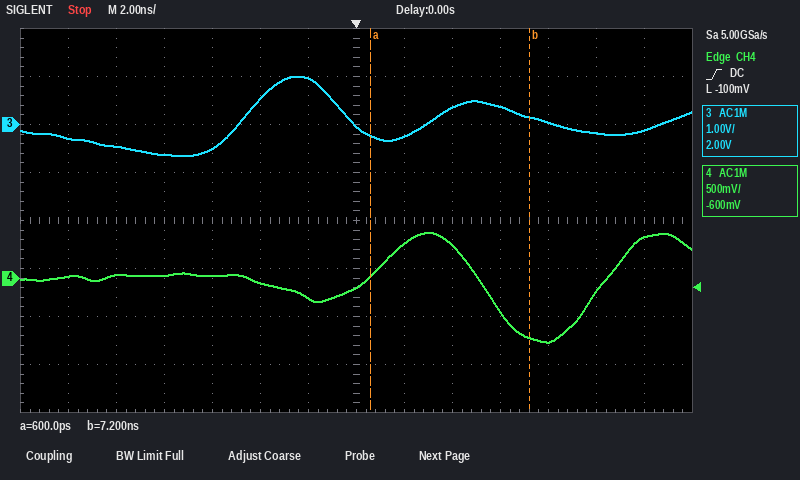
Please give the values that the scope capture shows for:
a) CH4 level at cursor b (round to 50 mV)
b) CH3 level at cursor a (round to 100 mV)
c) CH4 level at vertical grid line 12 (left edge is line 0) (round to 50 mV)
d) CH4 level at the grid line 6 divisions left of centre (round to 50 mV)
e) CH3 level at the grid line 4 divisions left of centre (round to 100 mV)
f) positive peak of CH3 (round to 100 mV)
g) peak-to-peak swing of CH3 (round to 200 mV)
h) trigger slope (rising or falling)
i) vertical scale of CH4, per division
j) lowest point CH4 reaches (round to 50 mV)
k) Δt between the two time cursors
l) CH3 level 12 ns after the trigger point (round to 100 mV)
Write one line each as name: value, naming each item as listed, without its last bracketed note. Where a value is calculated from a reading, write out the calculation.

CH4 level at cursor b: -600 mV
CH3 level at cursor a: -200 mV
CH4 level at vertical grid line 12 (left edge is line 0): -150 mV
CH4 level at the grid line 6 divisions left of centre: 0 mV
CH3 level at the grid line 4 divisions left of centre: -600 mV
positive peak of CH3: 1.0 V
peak-to-peak swing of CH3: 1.6 V
trigger slope: rising
vertical scale of CH4, per division: 500 mV
lowest point CH4 reaches: -650 mV
Δt between the two time cursors: 7.2 ns − (600 ps) = 6.6 ns
CH3 level 12 ns after the trigger point: -100 mV
